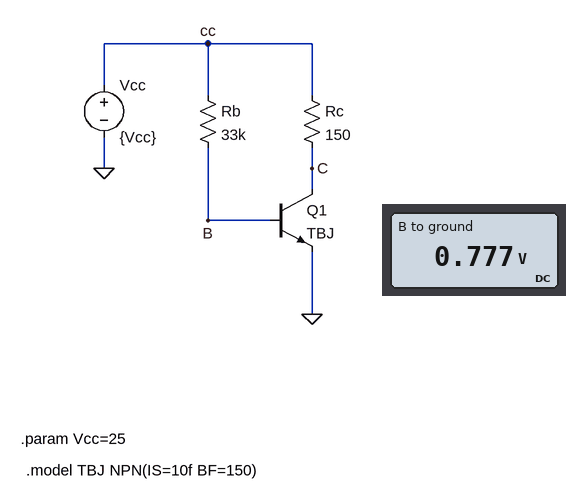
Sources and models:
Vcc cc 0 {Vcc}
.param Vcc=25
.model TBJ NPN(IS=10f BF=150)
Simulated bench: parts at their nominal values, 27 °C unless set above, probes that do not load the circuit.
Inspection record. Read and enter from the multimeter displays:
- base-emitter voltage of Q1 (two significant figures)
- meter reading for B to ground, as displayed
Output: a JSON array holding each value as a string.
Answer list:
["780 mV", "0.777 V"]
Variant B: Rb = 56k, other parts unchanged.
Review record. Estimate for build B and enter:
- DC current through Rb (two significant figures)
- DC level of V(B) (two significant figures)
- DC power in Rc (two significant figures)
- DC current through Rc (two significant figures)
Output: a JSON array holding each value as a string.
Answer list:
["430 µA", "760 mV", "630 mW", "65 mA"]
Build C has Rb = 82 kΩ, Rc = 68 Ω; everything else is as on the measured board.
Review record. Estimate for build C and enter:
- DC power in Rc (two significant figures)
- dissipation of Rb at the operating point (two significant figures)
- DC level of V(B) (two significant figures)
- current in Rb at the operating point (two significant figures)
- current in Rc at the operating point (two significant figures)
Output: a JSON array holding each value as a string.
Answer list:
["130 mW", "7.2 mW", "750 mV", "300 µA", "44 mA"]
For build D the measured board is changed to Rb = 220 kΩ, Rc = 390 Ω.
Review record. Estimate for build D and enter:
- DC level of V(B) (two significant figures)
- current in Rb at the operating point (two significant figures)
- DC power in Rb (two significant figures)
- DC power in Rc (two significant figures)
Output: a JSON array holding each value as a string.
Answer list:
["730 mV", "110 µA", "2.7 mW", "110 mW"]
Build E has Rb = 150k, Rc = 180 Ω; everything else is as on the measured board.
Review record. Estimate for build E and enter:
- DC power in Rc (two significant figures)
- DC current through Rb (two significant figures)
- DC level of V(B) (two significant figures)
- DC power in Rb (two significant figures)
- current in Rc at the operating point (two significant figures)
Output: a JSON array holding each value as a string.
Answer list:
["110 mW", "160 µA", "740 mV", "3.9 mW", "24 mA"]
